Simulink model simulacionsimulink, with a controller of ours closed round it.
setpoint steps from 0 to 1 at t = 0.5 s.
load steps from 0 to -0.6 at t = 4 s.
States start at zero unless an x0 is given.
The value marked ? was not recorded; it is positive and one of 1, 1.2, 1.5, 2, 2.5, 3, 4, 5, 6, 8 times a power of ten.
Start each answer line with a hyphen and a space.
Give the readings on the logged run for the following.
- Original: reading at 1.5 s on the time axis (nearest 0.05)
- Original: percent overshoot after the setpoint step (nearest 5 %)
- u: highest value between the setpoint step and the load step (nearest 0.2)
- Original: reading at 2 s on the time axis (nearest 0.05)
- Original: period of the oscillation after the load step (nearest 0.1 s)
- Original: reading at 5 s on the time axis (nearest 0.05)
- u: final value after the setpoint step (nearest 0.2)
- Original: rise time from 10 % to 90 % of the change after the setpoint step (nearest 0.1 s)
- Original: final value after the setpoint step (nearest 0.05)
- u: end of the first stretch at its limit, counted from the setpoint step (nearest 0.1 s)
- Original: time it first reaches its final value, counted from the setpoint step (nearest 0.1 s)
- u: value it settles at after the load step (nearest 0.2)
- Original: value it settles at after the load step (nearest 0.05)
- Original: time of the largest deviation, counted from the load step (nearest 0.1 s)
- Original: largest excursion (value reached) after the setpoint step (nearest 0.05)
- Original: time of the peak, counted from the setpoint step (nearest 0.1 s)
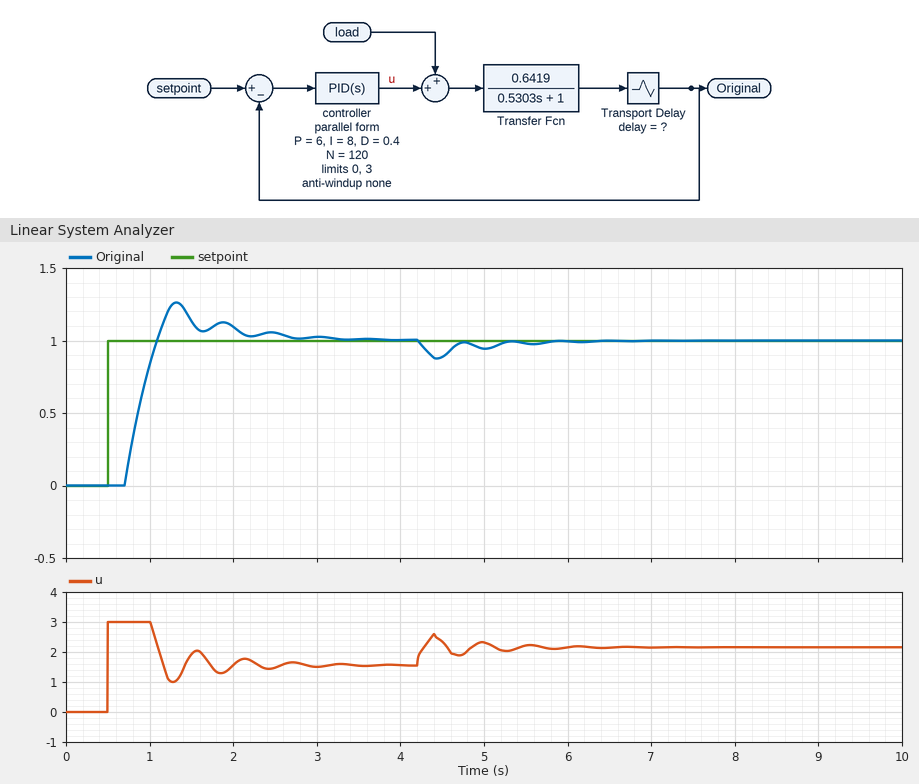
- 1.15
- 25 %
- 3.0
- 1.10
- 0.6 s
- 0.95
- 1.6
- 0.3 s
- 1.00
- 0.5 s
- 0.6 s
- 2.2
- 1.00
- 0.4 s
- 1.25
- 0.8 s
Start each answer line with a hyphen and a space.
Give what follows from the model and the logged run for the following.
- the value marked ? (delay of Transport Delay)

- 0.2
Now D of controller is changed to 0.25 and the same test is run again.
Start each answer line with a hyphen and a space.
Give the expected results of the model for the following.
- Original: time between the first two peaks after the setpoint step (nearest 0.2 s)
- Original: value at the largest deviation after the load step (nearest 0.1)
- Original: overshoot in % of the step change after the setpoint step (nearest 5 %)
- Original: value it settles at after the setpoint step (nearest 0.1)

- 0.6 s
- 0.9
- 30 %
- 1.0
